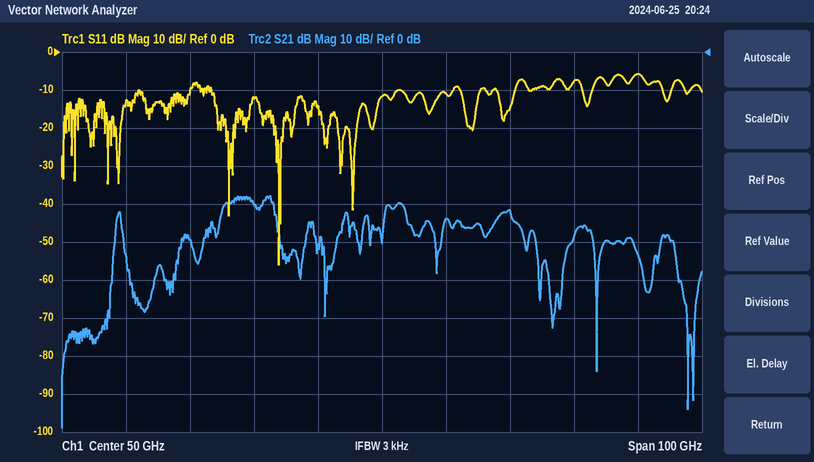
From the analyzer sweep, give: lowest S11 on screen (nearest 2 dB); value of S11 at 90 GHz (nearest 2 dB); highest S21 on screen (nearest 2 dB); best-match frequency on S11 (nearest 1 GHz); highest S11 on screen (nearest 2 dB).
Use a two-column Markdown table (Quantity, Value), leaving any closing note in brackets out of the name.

| Quantity | Value |
|---|---|
| lowest S11 on screen | -56 dB |
| value of S11 at 90 GHz | -6 dB |
| highest S21 on screen | -38 dB |
| best-match frequency on S11 | 34 GHz |
| highest S11 on screen | -6 dB |
